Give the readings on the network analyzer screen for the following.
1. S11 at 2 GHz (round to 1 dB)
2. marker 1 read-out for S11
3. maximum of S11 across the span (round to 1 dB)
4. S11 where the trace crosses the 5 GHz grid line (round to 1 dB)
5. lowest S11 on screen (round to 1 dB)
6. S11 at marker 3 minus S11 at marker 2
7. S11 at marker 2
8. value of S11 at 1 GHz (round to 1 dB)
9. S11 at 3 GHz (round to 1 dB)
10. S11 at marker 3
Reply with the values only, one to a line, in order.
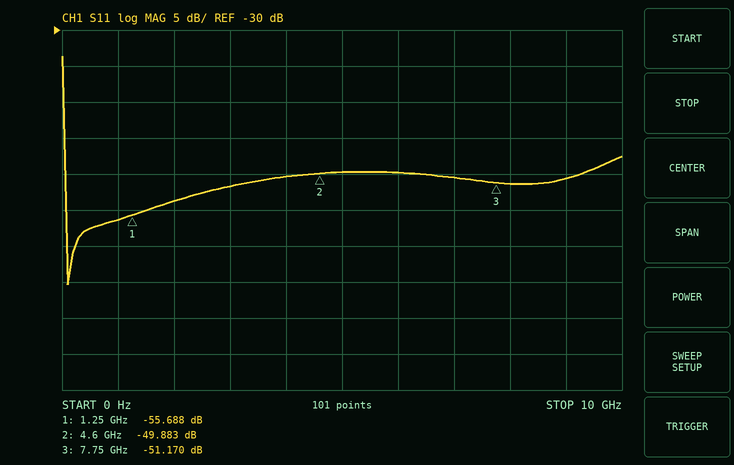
-54 dB
-55.688 dB
-34 dB
-50 dB
-65 dB
-1.287 dB
-49.883 dB
-56 dB
-52 dB
-51.170 dB
